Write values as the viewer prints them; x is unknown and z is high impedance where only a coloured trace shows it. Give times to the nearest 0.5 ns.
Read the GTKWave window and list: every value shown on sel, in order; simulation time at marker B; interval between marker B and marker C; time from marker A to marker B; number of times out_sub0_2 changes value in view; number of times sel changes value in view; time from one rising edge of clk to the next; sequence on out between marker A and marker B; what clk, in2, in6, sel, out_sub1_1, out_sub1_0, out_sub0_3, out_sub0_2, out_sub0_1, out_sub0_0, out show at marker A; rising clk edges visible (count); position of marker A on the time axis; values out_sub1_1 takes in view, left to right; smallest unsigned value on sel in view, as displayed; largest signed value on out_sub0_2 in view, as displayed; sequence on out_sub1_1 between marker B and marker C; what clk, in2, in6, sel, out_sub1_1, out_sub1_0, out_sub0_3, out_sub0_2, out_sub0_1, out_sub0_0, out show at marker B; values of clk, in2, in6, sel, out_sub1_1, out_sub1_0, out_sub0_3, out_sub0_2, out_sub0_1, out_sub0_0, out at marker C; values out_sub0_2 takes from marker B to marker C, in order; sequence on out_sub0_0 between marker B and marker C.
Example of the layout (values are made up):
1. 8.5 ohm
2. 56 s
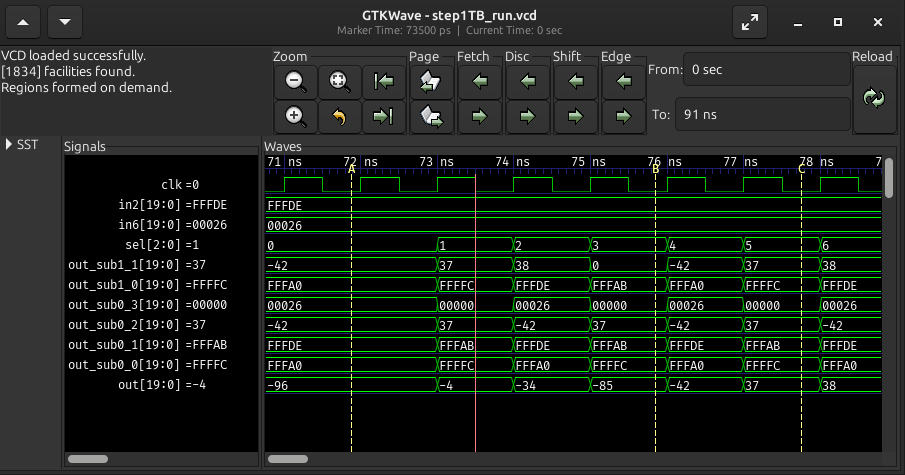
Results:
1. 0, 1, 2, 3, 4, 5, 6
2. 76 ns
3. 2 ns
4. 4 ns
5. 6
6. 6
7. 1 ns
8. -96, -4, -34, -85
9. clk=0, in2=FFFDE, in6=00026, sel=0, out_sub1_1=-42, out_sub1_0=FFFA0, out_sub0_3=00026, out_sub0_2=-42, out_sub0_1=FFFDE, out_sub0_0=FFFA0, out=-96
10. 8
11. 72 ns
12. -42, 37, 38, 0, -42, 37, 38
13. 0
14. 37
15. 0, -42, 37
16. clk=0, in2=FFFDE, in6=00026, sel=3, out_sub1_1=0, out_sub1_0=FFFAB, out_sub0_3=00000, out_sub0_2=37, out_sub0_1=FFFAB, out_sub0_0=FFFFC, out=-85
17. clk=0, in2=FFFDE, in6=00026, sel=5, out_sub1_1=37, out_sub1_0=FFFFC, out_sub0_3=00000, out_sub0_2=37, out_sub0_1=FFFAB, out_sub0_0=FFFFC, out=37
18. 37, -42, 37
19. FFFFC, FFFA0, FFFFC
